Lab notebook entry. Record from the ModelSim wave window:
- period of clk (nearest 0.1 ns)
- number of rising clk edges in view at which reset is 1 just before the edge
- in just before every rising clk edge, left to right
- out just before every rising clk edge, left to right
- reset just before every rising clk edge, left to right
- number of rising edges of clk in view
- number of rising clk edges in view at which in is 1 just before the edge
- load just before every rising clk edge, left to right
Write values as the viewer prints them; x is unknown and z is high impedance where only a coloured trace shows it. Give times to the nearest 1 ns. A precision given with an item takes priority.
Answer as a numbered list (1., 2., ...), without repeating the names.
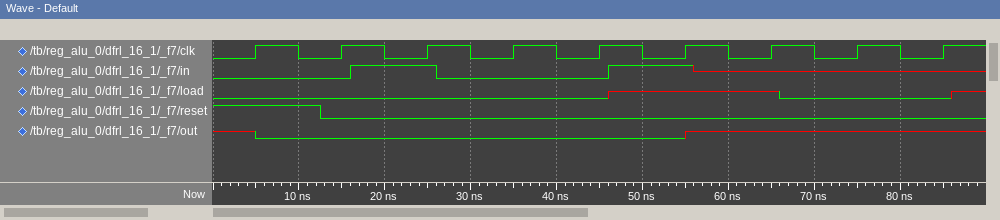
1. 10 ns
2. 1
3. 0 0 1 0 0 1 x x x
4. x 0 0 0 0 0 x x x
5. 1 0 0 0 0 0 0 0 0
6. 9
7. 2
8. 0 0 0 0 0 x x 0 0
